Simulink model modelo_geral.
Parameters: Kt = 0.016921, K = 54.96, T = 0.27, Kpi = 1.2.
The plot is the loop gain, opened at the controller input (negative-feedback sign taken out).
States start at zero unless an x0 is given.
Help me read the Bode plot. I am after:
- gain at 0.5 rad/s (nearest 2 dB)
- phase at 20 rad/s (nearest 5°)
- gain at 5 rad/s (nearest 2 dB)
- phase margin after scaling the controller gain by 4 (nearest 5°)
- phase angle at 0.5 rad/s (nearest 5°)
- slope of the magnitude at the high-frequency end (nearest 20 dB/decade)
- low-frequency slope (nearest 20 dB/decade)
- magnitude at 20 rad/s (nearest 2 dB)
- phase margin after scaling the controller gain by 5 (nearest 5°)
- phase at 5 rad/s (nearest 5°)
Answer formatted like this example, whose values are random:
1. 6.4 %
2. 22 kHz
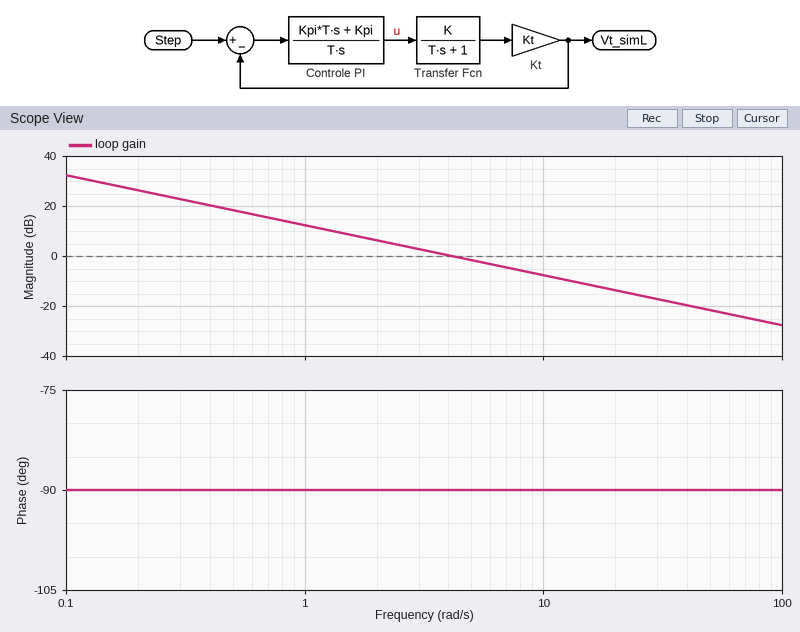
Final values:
1. 18 dB
2. -90°
3. -2 dB
4. 90°
5. -90°
6. -20 dB/decade
7. -20 dB/decade
8. -14 dB
9. 90°
10. -90°
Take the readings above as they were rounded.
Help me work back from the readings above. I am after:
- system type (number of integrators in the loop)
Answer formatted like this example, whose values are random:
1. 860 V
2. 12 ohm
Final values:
1. 1
